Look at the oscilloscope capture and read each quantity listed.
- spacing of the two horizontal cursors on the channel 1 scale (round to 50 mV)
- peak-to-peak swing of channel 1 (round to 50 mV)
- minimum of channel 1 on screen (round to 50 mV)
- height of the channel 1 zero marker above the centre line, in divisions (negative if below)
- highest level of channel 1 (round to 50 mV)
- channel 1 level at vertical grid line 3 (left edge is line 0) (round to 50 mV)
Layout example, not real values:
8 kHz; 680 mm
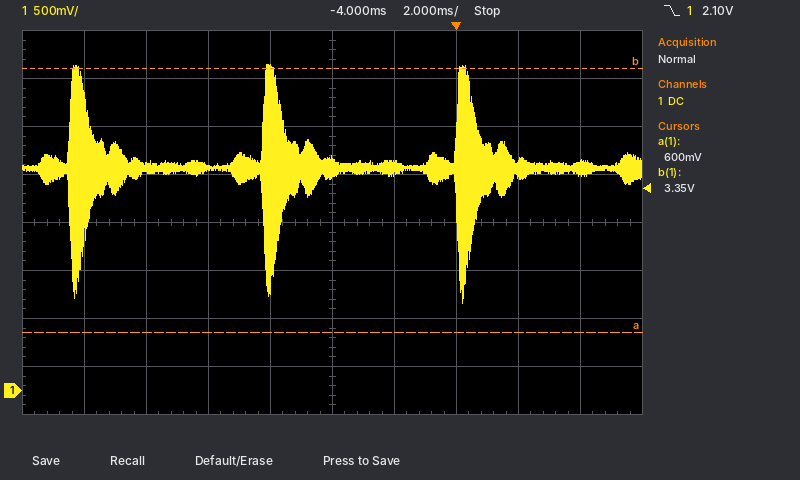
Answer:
2.75 V; 2.50 V; 900 mV; -3.5 div; 3.40 V; 2.30 V
